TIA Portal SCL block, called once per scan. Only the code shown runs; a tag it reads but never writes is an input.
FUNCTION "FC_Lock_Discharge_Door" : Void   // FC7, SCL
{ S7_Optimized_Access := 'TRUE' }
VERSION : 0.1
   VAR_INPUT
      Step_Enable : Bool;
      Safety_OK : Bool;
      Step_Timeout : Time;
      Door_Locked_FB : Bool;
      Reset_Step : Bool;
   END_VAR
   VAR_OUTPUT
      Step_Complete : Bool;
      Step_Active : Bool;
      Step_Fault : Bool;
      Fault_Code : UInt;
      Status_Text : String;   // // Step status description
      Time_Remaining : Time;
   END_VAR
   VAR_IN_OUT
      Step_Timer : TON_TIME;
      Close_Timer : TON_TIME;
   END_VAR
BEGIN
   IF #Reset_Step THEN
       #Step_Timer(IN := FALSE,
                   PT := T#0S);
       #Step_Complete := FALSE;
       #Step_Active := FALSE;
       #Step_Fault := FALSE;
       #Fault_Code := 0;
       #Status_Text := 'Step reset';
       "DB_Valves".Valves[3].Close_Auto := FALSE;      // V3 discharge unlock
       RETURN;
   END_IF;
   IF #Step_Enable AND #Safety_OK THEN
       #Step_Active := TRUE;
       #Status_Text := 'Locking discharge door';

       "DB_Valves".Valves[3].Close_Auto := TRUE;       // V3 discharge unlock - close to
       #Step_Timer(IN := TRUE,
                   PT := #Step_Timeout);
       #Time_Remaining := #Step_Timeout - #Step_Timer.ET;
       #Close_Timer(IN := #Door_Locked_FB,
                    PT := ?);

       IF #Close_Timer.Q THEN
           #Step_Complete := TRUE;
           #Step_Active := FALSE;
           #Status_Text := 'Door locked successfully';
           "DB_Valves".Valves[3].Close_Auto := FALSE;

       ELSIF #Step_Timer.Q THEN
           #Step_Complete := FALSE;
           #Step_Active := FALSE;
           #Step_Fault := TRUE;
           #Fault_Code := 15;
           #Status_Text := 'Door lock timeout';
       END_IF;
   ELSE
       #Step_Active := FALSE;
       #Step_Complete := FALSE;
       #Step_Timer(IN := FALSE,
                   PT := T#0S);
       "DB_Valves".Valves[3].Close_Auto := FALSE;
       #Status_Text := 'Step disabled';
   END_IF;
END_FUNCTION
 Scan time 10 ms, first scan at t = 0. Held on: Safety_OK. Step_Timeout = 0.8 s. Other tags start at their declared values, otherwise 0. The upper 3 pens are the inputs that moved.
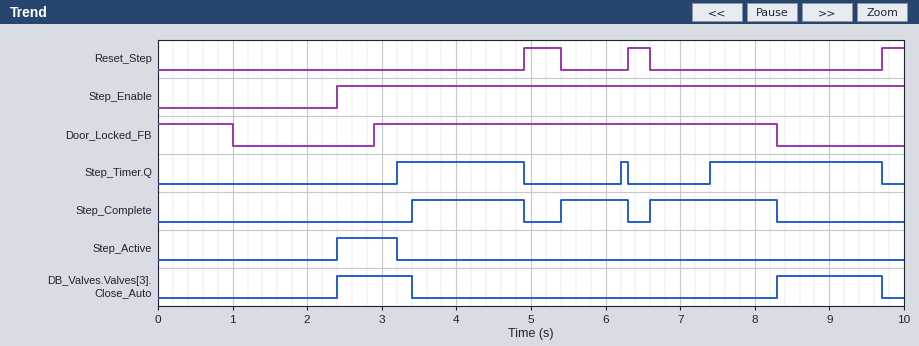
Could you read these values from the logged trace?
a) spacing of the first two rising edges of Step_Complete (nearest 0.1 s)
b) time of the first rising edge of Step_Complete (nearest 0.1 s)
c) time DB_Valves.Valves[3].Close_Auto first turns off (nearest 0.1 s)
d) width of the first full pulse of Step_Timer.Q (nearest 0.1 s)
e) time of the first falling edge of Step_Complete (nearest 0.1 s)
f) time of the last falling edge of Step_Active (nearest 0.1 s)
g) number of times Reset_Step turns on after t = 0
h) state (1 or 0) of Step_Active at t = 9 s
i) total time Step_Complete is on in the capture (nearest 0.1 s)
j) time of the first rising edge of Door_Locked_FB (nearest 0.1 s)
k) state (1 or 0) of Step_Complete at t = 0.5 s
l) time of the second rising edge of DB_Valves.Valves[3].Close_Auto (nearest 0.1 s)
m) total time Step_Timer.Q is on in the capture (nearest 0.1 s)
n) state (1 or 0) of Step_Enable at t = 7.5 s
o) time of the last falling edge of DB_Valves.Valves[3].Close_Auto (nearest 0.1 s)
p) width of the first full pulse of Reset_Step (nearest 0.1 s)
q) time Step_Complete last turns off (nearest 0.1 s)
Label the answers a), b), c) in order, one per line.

a) 2.0 s
b) 3.4 s
c) 3.4 s
d) 1.7 s
e) 4.9 s
f) 3.2 s
g) 3
h) 0
i) 4.1 s
j) 2.9 s
k) 0
l) 8.3 s
m) 4.1 s
n) 1
o) 9.7 s
p) 0.5 s
q) 8.3 s
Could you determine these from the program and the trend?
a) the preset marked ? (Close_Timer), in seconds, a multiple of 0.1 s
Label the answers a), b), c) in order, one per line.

a) 0.5 s
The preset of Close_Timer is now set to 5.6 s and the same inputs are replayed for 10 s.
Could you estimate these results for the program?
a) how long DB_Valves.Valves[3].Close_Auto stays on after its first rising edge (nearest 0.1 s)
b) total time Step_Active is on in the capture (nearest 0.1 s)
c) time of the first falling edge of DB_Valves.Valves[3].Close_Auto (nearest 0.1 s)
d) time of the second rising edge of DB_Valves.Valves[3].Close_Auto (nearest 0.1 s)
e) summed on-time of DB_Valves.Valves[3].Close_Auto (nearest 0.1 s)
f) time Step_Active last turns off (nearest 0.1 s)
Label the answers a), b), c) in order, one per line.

a) 2.5 s
b) 2.4 s
c) 4.9 s
d) 5.4 s
e) 6.5 s
f) 7.4 s
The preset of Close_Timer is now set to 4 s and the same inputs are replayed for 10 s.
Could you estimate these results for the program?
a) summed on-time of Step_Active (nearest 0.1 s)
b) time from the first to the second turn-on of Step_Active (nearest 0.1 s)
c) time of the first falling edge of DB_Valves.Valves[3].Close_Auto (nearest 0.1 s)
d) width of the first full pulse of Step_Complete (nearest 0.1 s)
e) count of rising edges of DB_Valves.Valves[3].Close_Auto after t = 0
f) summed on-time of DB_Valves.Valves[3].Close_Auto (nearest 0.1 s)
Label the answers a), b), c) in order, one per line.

a) 1.9 s
b) 3.0 s
c) 4.9 s
d) 1.4 s
e) 4
f) 5.1 s
